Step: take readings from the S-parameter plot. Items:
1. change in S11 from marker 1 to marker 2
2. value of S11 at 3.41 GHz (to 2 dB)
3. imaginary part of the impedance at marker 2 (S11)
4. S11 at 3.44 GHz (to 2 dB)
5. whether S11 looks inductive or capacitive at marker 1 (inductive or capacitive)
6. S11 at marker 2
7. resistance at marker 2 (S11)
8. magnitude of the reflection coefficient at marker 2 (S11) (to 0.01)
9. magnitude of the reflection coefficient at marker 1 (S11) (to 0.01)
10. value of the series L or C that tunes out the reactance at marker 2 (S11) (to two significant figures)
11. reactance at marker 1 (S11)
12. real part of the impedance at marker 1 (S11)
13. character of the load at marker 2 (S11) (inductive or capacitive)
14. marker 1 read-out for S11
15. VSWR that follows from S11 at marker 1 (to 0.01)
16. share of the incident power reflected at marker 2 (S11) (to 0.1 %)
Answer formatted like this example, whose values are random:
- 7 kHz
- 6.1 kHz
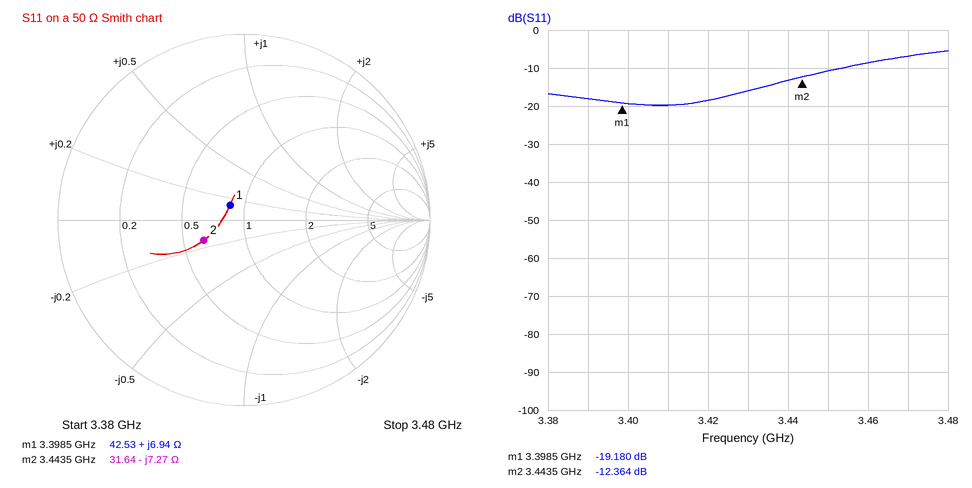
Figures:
- 6.816 dB
- -20 dB
- -7.27 Ω
- -14 dB
- inductive
- -12.364 dB
- 31.64 Ω
- 0.24
- 0.11
- 340 pH
- +6.94 Ω
- 42.53 Ω
- capacitive
- -19.180 dB
- 1.25
- 5.8 %
